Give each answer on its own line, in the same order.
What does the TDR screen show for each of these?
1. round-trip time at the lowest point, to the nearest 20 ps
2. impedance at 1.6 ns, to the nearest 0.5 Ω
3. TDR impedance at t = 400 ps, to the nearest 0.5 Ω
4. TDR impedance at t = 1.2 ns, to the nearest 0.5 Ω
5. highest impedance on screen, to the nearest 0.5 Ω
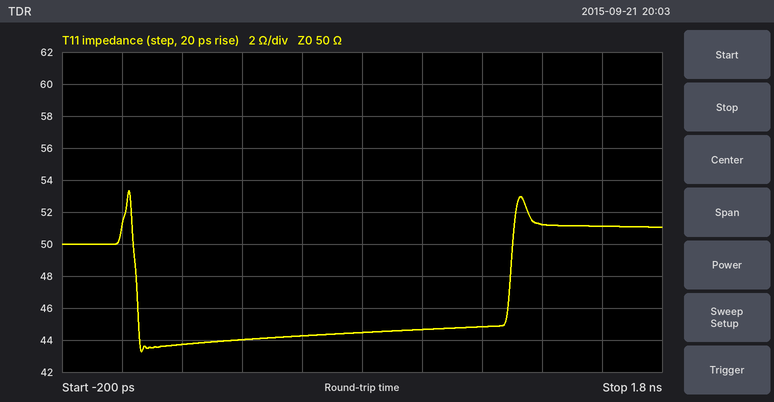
60 ps
51.0 Ω
44.0 Ω
45.0 Ω
53.5 Ω
